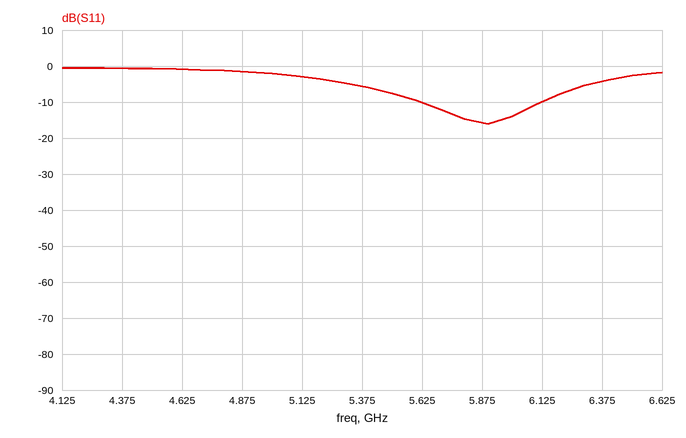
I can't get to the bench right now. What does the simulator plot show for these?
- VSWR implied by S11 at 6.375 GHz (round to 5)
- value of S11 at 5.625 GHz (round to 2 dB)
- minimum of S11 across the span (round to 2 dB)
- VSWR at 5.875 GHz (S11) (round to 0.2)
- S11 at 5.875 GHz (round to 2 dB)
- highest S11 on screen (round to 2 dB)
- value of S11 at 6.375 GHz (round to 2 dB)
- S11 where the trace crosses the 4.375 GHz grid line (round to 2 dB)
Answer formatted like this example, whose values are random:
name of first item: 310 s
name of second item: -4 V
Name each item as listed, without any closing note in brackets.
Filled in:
VSWR implied by S11 at 6.375 GHz: 5
value of S11 at 5.625 GHz: -10 dB
minimum of S11 across the span: -16 dB
VSWR at 5.875 GHz (S11): 1.4
S11 at 5.875 GHz: -16 dB
highest S11 on screen: 0 dB
value of S11 at 6.375 GHz: -4 dB
S11 where the trace crosses the 4.375 GHz grid line: 0 dB
